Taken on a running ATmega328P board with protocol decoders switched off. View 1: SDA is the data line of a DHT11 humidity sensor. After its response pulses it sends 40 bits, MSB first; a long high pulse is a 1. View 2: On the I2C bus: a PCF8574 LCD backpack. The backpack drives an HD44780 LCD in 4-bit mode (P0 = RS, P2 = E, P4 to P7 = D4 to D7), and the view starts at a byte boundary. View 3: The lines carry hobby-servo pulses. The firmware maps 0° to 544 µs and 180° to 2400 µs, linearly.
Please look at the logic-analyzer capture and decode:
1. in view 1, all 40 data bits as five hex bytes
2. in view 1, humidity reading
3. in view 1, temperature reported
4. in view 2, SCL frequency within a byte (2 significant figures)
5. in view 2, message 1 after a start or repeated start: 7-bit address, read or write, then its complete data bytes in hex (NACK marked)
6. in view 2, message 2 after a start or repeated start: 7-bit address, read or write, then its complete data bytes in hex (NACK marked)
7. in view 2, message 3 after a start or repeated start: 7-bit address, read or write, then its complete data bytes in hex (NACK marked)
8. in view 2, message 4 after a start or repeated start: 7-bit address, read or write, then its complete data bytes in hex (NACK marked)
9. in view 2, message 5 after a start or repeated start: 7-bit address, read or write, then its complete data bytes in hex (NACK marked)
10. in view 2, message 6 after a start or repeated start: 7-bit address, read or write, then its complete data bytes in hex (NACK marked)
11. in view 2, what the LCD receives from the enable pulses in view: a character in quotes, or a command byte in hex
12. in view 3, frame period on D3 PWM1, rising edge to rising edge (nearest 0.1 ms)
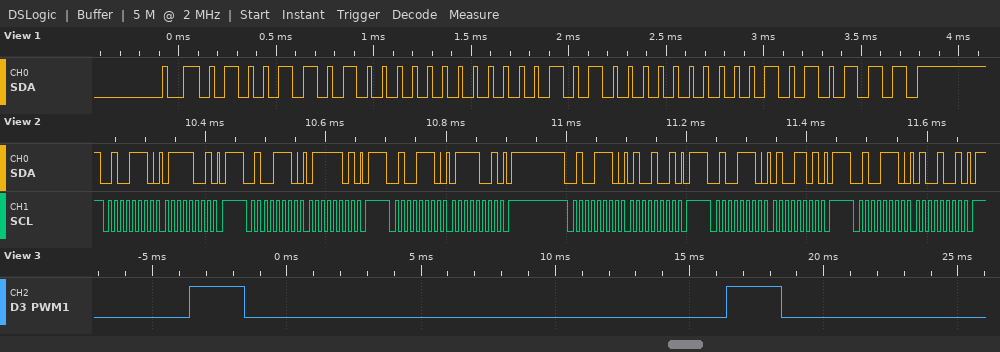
4D 00 0A 00 57
77 %
10.0 °C
100 kHz
0x27 write: 79
0x27 write: 7D
0x27 write: 79
0x27 write: 49
0x27 write: 4D
0x27 write: 49
't'
20.0 ms
